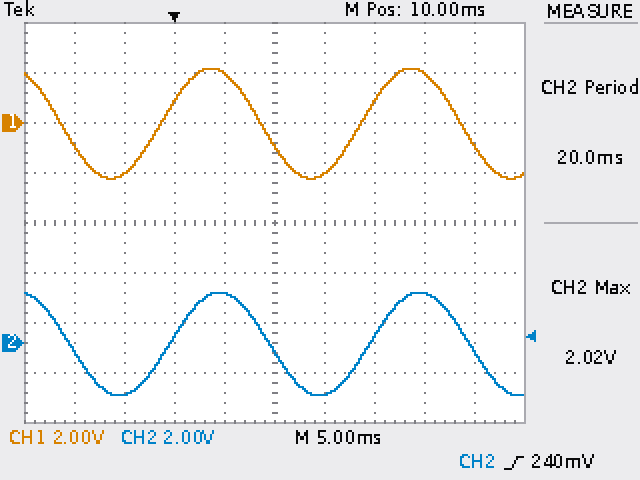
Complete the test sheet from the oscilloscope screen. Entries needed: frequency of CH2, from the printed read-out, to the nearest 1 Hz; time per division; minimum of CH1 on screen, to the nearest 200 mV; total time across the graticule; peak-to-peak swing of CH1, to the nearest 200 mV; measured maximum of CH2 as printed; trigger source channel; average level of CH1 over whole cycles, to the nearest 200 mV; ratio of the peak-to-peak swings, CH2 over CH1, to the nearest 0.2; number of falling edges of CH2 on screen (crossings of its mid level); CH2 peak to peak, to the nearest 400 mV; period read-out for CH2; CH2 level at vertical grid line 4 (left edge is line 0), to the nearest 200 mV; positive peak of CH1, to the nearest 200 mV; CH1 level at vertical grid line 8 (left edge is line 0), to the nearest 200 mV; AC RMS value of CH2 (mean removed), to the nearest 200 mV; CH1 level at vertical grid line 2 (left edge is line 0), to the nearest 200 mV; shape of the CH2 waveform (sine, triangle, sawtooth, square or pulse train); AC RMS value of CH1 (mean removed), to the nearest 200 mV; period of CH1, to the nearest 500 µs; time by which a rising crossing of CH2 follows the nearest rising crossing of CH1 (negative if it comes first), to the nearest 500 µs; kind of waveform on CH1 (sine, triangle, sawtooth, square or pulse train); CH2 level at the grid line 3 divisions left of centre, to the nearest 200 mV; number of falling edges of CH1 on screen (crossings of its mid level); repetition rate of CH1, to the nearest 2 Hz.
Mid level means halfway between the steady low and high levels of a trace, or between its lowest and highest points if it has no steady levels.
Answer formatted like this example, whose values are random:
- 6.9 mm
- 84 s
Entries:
- 50 Hz
- 5 ms
- -2.2 V
- 50 ms
- 4.4 V
- 2.02 V
- CH2
- 0.0 V
- 1.0
- 3
- 4.0 V
- 20.0 ms
- 2.0 V
- 2.2 V
- 2.0 V
- 1.4 V
- -2.0 V
- sine
- 1.6 V
- 20.0 ms
- +1.0 ms
- sine
- -2.0 V
- 3
- 50 Hz
